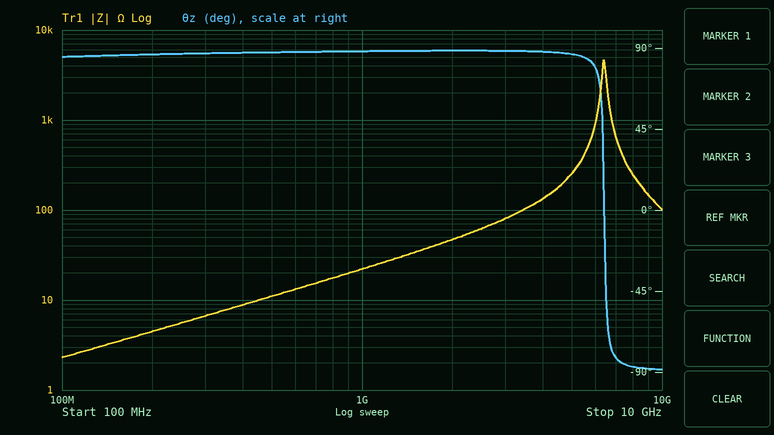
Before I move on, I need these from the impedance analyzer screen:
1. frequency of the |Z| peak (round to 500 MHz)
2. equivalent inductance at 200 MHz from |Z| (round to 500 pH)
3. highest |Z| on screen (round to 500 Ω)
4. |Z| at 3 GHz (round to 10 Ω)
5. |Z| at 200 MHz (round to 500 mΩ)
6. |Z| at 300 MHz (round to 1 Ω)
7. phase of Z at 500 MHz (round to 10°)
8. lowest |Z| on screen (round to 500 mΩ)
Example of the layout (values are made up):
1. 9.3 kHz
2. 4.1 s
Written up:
1. 6.5 GHz
2. 3.5 nH
3. 4.5 kΩ
4. 80 Ω
5. 4.5 Ω
6. 7 Ω
7. 90°
8. 2.5 Ω
